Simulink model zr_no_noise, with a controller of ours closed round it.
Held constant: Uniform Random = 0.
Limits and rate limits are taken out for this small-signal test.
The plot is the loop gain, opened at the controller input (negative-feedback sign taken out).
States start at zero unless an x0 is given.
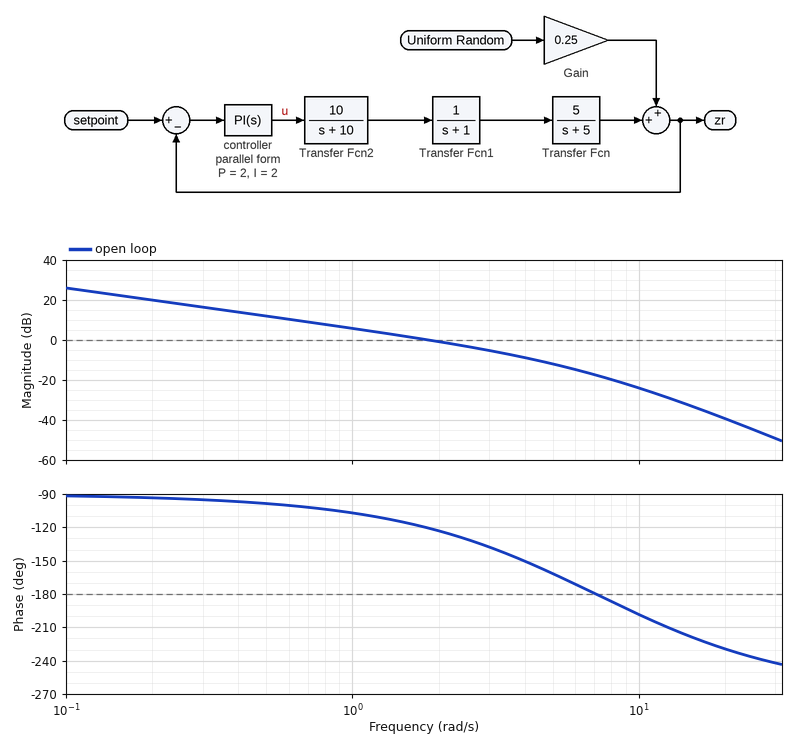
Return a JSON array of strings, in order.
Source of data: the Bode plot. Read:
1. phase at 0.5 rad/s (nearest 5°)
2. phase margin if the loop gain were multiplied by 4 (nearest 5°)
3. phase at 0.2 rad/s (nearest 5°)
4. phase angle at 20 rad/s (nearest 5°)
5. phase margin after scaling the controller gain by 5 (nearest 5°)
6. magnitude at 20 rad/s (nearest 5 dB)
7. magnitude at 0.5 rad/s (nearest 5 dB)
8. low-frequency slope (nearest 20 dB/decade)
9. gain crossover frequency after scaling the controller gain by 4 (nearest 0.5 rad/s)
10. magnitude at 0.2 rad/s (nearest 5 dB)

["-100°", "20°", "-95°", "-230°", "10°", "-40 dB", "10 dB", "-20 dB/decade", "5.0 rad/s", "20 dB"]
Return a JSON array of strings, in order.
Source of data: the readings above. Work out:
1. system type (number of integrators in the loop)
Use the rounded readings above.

["1"]
